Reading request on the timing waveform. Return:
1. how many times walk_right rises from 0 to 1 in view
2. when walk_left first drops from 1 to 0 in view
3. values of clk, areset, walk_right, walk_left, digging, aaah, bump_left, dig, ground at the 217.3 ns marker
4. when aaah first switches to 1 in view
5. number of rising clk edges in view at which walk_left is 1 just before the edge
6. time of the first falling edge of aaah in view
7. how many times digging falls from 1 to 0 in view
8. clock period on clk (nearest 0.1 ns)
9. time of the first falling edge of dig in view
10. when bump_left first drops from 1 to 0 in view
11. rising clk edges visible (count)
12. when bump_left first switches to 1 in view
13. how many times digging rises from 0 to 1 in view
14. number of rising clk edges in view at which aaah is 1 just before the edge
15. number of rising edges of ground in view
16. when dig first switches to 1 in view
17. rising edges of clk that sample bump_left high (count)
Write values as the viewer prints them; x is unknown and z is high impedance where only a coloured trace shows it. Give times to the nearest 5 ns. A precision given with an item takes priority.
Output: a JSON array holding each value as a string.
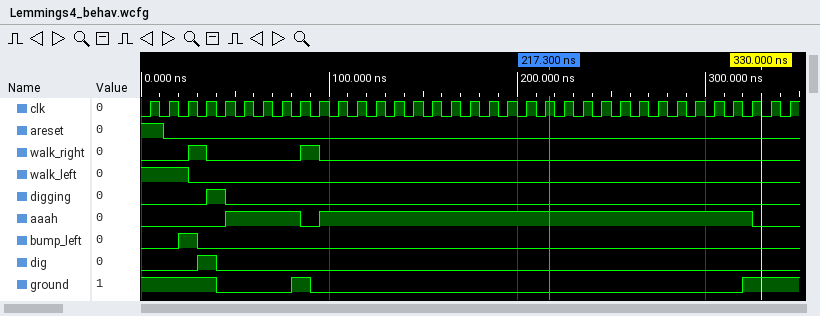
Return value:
["2", "25 ns", "clk=1, areset=0, walk_right=0, walk_left=0, digging=0, aaah=1, bump_left=0, dig=0, ground=0", "45 ns", "3", "85 ns", "1", "10 ns", "40 ns", "30 ns", "35", "20 ns", "1", "27", "2", "30 ns", "1"]
